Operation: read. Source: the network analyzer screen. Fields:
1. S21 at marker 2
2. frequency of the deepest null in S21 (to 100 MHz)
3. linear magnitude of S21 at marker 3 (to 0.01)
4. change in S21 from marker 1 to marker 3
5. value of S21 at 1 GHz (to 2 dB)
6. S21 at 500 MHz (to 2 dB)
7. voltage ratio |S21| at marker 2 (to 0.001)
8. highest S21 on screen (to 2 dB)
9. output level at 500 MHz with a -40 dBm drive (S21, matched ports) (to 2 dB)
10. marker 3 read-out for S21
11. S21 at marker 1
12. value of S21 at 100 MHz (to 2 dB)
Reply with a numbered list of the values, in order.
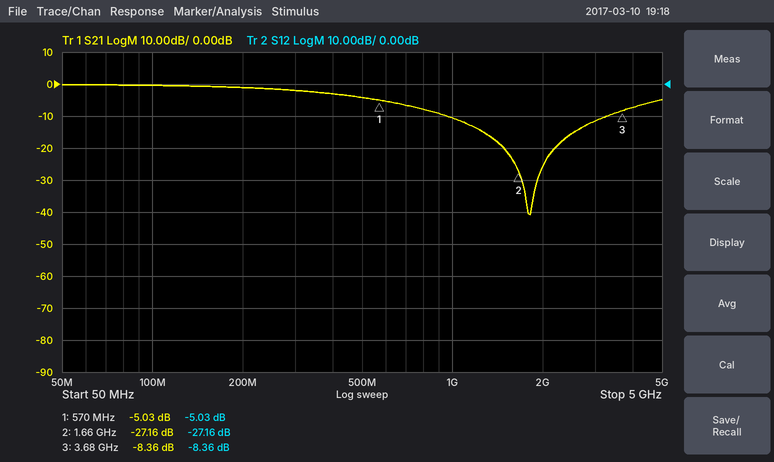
1. -27.16 dB
2. 1.8 GHz
3. 0.38
4. -3.33 dB
5. -10 dB
6. -4 dB
7. 0.044
8. 0 dB
9. -44 dBm
10. -8.36 dB
11. -5.03 dB
12. 0 dB
